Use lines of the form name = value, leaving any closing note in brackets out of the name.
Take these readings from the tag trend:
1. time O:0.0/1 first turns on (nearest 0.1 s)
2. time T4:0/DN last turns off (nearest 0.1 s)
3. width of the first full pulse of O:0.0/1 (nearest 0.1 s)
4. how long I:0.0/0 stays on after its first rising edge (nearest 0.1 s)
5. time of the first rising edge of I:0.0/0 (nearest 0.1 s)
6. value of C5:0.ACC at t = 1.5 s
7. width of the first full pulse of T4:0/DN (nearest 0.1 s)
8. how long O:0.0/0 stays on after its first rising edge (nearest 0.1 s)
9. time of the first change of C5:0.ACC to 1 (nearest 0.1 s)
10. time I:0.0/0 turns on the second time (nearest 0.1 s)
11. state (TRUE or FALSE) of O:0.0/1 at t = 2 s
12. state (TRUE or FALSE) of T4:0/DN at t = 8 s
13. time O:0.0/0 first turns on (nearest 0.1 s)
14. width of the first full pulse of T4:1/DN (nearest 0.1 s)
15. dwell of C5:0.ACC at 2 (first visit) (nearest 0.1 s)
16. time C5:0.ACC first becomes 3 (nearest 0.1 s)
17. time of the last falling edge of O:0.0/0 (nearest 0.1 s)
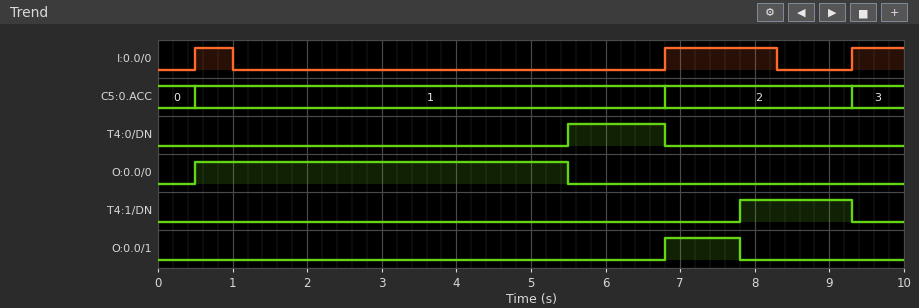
time O:0.0/1 first turns on = 6.8 s
time T4:0/DN last turns off = 6.8 s
width of the first full pulse of O:0.0/1 = 1.0 s
how long I:0.0/0 stays on after its first rising edge = 0.5 s
time of the first rising edge of I:0.0/0 = 0.5 s
value of C5:0.ACC at t = 1.5 s = 1
width of the first full pulse of T4:0/DN = 1.3 s
how long O:0.0/0 stays on after its first rising edge = 5.0 s
time of the first change of C5:0.ACC to 1 = 0.5 s
time I:0.0/0 turns on the second time = 6.8 s
state (TRUE or FALSE) of O:0.0/1 at t = 2 s = FALSE
state (TRUE or FALSE) of T4:0/DN at t = 8 s = FALSE
time O:0.0/0 first turns on = 0.5 s
width of the first full pulse of T4:1/DN = 1.5 s
dwell of C5:0.ACC at 2 (first visit) = 2.5 s
time C5:0.ACC first becomes 3 = 9.3 s
time of the last falling edge of O:0.0/0 = 5.5 s
